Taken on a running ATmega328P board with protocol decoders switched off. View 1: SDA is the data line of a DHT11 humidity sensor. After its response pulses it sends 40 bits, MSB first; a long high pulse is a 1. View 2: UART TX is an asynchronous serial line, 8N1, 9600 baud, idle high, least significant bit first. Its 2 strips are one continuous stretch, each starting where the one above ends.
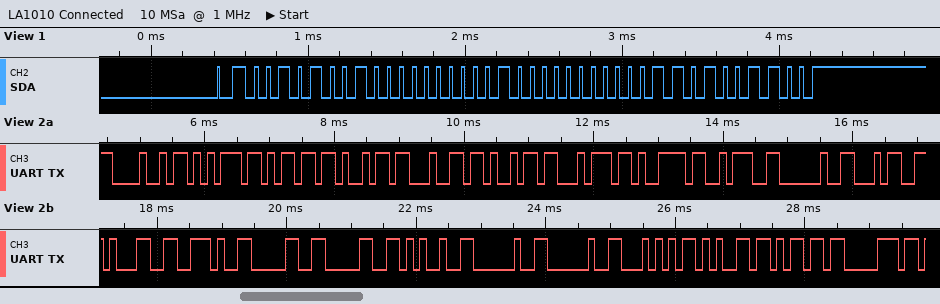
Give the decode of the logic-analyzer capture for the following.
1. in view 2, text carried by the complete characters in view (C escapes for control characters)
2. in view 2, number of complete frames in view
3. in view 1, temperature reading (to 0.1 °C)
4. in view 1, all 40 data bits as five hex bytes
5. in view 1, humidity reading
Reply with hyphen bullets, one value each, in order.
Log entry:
- "Humidity: 41.00%  Temp"
- 22
- 32.3 °C
- 29 00 20 03 4C
- 41 %
